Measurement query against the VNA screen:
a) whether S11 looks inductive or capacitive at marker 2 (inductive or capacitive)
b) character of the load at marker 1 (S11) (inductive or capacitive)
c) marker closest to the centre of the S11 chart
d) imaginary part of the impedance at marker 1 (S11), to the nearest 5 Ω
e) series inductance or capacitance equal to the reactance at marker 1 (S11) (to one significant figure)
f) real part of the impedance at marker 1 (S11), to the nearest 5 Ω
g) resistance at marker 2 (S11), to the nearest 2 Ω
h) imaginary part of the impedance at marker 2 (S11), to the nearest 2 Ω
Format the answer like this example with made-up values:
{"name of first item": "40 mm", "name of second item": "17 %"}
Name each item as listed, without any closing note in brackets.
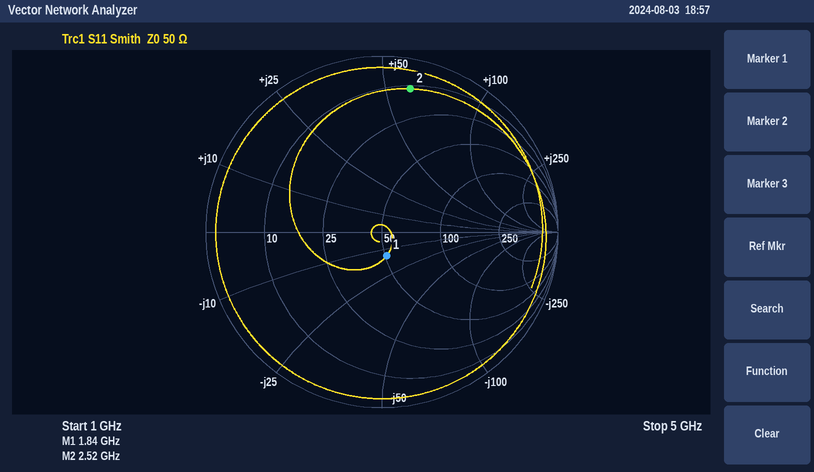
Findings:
{"whether S11 looks inductive or capacitive at marker 2": "inductive", "character of the load at marker 1 (S11)": "capacitive", "marker closest to the centre of the S11 chart": "marker 1", "imaginary part of the impedance at marker 1 (S11), to the nearest 5 Ω": "-15 Ω", "series inductance or capacitance equal to the reactance at marker 1 (S11)": "6 pF", "real part of the impedance at marker 1 (S11), to the nearest 5 Ω": "50 Ω", "resistance at marker 2 (S11), to the nearest 2 Ω": "12 Ω", "imaginary part of the impedance at marker 2 (S11), to the nearest 2 Ω": "+60 Ω"}
